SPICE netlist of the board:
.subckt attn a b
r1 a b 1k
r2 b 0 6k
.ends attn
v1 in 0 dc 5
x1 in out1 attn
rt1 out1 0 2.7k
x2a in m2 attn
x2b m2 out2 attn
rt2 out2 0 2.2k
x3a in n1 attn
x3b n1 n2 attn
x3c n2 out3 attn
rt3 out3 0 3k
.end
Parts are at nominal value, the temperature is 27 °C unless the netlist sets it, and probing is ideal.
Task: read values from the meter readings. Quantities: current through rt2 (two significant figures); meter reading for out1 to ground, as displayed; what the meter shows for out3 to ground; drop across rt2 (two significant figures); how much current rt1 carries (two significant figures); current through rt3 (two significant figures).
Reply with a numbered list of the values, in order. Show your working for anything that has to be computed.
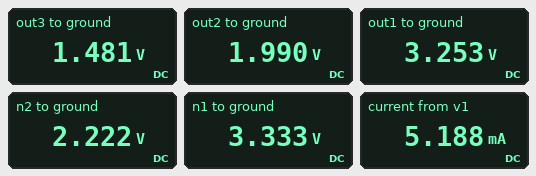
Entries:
1. (1.99 V) / 2.2 kΩ = 900 µA
2. 3.253 V
3. 1.481 V
4. 1.99 V = 2.0 V
5. (3.253 V) / 2.7 kΩ = 1.2 mA
6. (1.481 V) / 3 kΩ = 490 µA
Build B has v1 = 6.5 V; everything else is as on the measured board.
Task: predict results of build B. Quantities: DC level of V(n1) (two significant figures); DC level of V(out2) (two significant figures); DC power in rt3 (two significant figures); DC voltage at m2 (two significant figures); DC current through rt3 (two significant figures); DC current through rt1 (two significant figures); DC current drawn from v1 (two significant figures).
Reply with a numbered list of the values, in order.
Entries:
1. 4.3 V
2. 2.6 V
3. 1.2 mW
4. 4.2 V
5. 640 µA
6. 1.6 mA
7. 6.7 mA
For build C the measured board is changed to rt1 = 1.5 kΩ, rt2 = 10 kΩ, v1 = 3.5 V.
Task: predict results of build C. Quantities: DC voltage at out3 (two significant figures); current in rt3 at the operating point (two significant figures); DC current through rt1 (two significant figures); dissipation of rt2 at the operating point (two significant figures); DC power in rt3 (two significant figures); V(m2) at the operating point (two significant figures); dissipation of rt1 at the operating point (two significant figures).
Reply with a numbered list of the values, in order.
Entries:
1. 1.0 V
2. 350 µA
3. 1.3 mA
4. 400 µW
5. 360 µW
6. 2.5 V
7. 2.4 mW
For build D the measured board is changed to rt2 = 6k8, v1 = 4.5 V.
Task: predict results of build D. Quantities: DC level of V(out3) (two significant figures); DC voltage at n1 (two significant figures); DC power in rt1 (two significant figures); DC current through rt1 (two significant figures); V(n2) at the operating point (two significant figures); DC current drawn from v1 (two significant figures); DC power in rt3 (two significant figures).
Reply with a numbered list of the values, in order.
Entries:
1. 1.3 V
2. 3.0 V
3. 3.2 mW
4. 1.1 mA
5. 2.0 V
6. 4.4 mA
7. 590 µW
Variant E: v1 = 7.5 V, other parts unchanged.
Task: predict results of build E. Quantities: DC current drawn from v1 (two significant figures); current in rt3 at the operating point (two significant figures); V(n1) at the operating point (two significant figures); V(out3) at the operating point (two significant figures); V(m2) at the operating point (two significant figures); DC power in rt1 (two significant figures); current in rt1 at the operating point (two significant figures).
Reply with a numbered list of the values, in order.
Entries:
1. 7.8 mA
2. 740 µA
3. 5.0 V
4. 2.2 V
5. 4.8 V
6. 8.8 mW
7. 1.8 mA
